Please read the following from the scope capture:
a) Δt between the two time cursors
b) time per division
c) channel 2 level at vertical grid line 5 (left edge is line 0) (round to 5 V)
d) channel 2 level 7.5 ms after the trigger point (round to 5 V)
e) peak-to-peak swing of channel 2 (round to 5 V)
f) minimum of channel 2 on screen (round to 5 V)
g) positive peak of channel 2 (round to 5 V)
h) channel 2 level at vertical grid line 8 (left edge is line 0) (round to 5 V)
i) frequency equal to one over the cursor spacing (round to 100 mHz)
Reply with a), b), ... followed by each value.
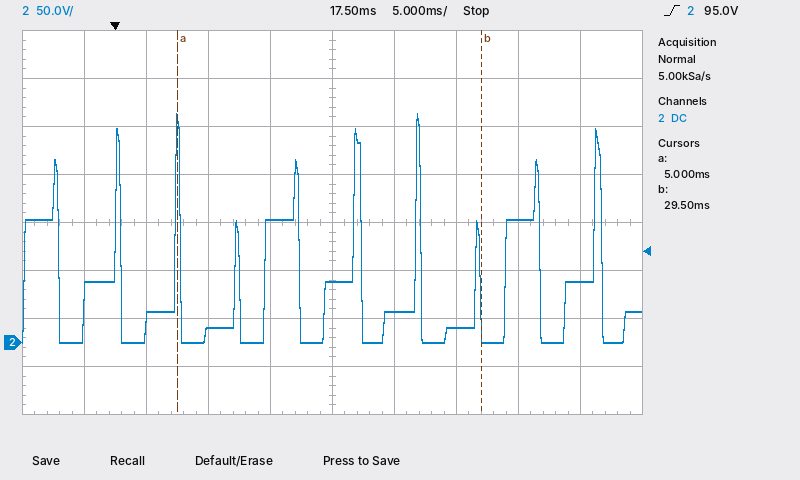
a) 24.5 ms
b) 5 ms
c) 65 V
d) 10 V
e) 240 V
f) 0 V
g) 240 V
h) 130 V
i) 40.8 Hz
